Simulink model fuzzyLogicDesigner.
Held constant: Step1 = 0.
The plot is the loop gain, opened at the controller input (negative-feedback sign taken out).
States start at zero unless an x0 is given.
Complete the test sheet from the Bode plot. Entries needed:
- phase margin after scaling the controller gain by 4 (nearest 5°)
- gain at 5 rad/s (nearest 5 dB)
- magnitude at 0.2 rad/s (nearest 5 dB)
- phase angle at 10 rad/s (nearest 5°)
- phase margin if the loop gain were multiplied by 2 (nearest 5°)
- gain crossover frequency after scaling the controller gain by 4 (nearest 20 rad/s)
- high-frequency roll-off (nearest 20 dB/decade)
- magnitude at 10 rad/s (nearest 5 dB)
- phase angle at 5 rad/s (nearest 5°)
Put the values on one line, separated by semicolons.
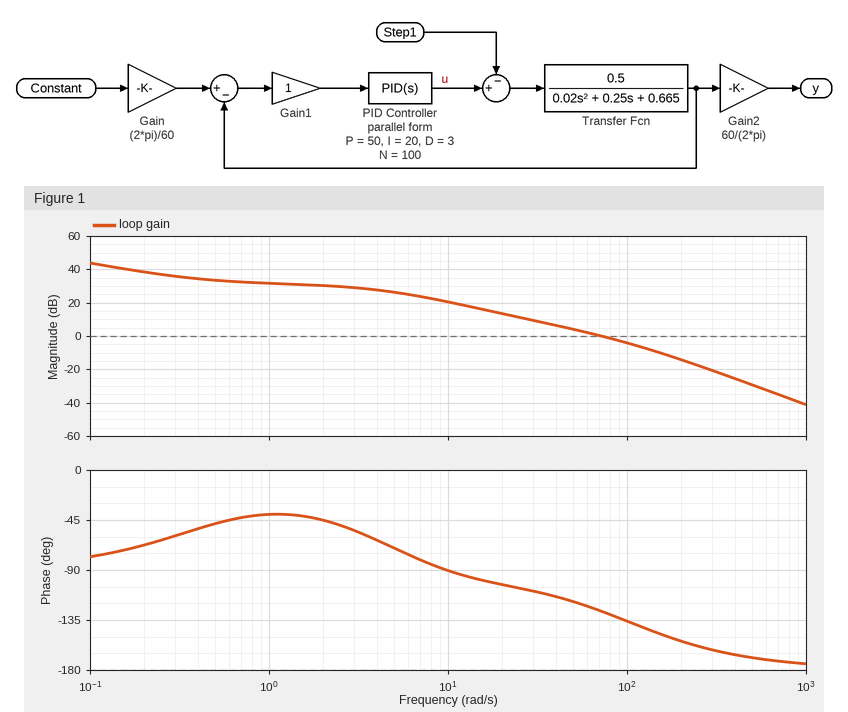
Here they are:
30°; 25 dB; 40 dB; -90°; 40°; 180 rad/s; -40 dB/decade; 20 dB; -70°
